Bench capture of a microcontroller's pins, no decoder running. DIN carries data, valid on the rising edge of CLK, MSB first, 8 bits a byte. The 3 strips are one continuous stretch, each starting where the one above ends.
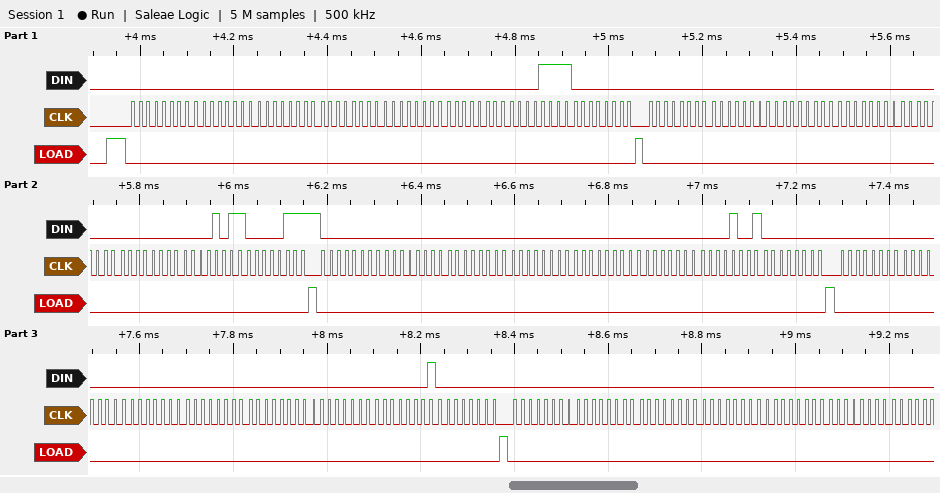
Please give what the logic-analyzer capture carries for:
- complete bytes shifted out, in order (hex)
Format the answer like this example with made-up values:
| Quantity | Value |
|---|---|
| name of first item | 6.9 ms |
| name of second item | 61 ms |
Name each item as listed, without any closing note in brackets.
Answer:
| Quantity | Value |
|---|---|
| complete bytes shifted out, in order | 00 00 00 00 00 00 0F 00 00 00 00 00 00 00 0B 07 00 00 00 00 00 00 09 00 00 00 00 00 00 00 01 00 00 00 00 00 00 00 |
